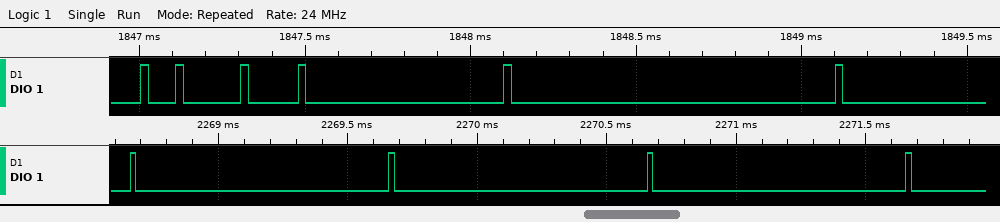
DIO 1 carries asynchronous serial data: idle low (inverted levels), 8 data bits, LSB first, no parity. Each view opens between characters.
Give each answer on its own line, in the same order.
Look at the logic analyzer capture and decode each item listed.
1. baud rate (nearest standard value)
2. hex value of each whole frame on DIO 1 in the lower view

38400 baud
FF, FF, FF, FF
